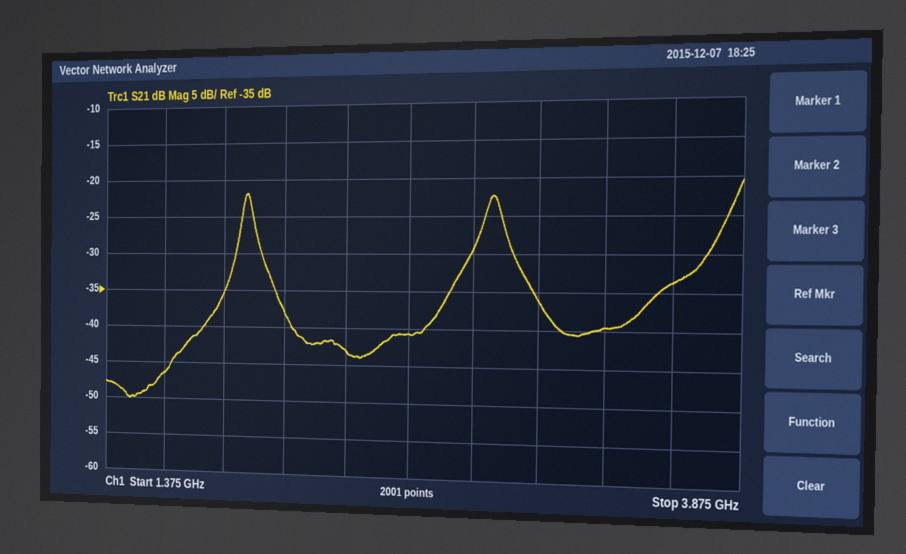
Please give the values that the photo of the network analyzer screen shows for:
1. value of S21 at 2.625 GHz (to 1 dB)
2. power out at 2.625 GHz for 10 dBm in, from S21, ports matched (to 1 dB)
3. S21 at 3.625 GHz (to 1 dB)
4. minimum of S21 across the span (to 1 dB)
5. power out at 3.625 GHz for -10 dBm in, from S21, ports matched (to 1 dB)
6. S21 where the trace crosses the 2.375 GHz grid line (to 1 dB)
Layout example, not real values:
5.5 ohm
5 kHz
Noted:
-41 dB
-31 dBm
-34 dB
-50 dB
-44 dBm
-43 dB
